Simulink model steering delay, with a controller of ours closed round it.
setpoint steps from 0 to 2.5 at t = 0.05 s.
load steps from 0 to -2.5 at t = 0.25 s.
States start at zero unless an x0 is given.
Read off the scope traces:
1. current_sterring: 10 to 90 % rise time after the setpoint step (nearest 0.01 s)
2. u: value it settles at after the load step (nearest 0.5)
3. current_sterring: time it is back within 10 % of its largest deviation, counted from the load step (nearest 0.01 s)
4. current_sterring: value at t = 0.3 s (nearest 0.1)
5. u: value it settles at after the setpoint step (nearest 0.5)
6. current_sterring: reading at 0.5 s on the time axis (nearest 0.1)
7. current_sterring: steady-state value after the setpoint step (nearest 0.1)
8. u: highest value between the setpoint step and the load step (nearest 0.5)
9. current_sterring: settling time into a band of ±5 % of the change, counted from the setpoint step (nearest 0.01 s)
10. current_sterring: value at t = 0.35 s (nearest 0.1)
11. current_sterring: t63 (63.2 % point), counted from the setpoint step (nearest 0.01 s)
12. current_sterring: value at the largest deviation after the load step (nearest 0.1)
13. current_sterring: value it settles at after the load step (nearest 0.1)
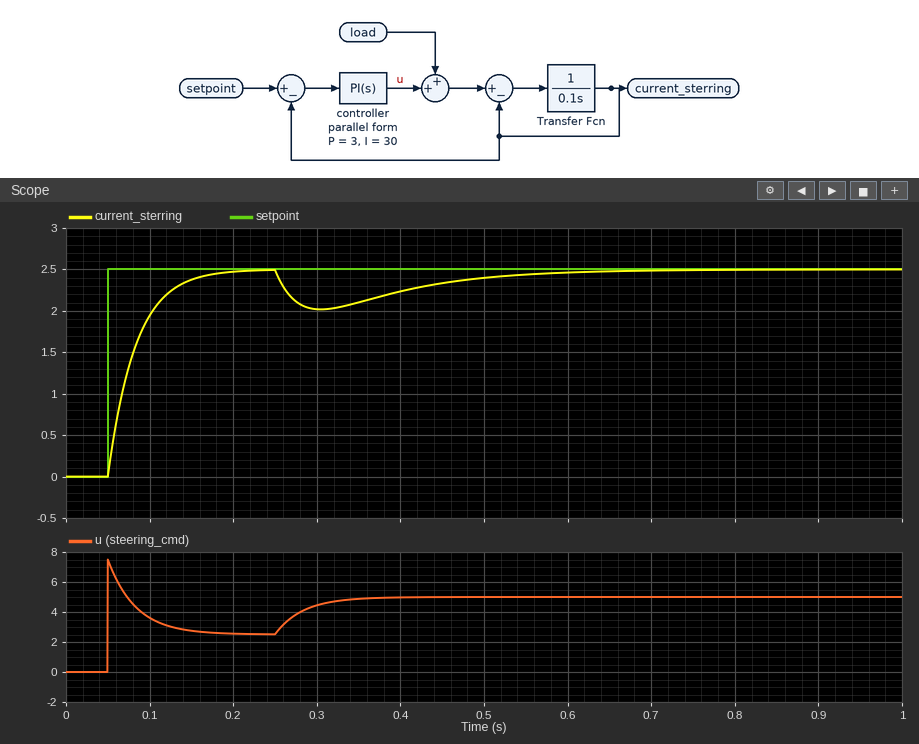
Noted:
0.07 s
5.0
0.33 s
2.0
2.5
2.4
2.5
7.5
0.10 s
2.1
0.03 s
2.0
2.5
